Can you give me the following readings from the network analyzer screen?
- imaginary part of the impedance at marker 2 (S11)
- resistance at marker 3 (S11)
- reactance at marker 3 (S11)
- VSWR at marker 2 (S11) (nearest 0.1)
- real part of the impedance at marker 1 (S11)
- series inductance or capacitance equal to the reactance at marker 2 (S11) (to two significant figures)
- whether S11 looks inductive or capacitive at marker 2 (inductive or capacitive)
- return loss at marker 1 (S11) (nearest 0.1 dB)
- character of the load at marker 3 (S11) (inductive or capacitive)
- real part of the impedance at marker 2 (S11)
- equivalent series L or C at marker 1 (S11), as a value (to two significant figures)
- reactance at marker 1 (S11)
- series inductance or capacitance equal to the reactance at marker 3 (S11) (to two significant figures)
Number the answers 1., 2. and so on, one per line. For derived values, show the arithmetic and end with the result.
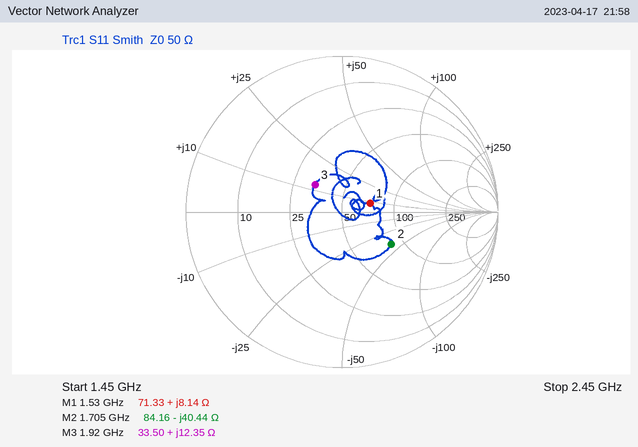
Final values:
1. -40.44 Ω
2. 33.50 Ω
3. +12.35 Ω
4. 2.2
5. 71.33 Ω
6. C = 1/(2π × 1.705 GHz × 40.44 Ω) ≈ 2.3 pF
7. capacitive
8. 14.5 dB
9. inductive
10. 84.16 Ω
11. L = 8.14 Ω/(2π × 1.53 GHz) ≈ 847 pH, so 850 pH to two significant figures
12. +8.14 Ω
13. L = 12.35 Ω/(2π × 1.92 GHz) ≈ 1.0 nH
